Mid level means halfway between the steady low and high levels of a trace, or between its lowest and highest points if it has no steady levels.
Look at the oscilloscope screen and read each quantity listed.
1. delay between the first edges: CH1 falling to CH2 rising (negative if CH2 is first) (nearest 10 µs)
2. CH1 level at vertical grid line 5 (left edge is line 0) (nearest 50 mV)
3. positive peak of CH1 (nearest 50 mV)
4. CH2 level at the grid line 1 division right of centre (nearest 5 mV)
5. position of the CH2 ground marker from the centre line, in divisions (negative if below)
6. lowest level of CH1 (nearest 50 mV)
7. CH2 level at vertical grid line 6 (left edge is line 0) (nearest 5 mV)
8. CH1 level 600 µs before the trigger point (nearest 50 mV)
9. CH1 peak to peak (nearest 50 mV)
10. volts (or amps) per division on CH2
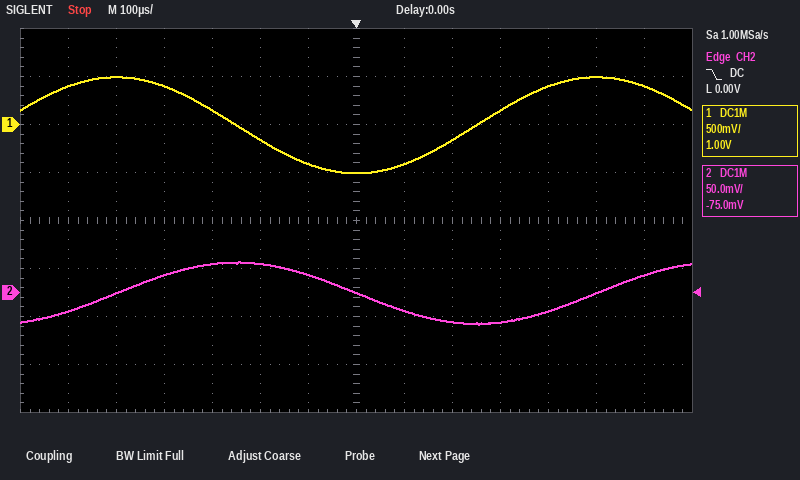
-250 µs
-150 mV
500 mV
-20 mV
-1.5 div
-500 mV
20 mV
400 mV
1.00 V
50 mV
